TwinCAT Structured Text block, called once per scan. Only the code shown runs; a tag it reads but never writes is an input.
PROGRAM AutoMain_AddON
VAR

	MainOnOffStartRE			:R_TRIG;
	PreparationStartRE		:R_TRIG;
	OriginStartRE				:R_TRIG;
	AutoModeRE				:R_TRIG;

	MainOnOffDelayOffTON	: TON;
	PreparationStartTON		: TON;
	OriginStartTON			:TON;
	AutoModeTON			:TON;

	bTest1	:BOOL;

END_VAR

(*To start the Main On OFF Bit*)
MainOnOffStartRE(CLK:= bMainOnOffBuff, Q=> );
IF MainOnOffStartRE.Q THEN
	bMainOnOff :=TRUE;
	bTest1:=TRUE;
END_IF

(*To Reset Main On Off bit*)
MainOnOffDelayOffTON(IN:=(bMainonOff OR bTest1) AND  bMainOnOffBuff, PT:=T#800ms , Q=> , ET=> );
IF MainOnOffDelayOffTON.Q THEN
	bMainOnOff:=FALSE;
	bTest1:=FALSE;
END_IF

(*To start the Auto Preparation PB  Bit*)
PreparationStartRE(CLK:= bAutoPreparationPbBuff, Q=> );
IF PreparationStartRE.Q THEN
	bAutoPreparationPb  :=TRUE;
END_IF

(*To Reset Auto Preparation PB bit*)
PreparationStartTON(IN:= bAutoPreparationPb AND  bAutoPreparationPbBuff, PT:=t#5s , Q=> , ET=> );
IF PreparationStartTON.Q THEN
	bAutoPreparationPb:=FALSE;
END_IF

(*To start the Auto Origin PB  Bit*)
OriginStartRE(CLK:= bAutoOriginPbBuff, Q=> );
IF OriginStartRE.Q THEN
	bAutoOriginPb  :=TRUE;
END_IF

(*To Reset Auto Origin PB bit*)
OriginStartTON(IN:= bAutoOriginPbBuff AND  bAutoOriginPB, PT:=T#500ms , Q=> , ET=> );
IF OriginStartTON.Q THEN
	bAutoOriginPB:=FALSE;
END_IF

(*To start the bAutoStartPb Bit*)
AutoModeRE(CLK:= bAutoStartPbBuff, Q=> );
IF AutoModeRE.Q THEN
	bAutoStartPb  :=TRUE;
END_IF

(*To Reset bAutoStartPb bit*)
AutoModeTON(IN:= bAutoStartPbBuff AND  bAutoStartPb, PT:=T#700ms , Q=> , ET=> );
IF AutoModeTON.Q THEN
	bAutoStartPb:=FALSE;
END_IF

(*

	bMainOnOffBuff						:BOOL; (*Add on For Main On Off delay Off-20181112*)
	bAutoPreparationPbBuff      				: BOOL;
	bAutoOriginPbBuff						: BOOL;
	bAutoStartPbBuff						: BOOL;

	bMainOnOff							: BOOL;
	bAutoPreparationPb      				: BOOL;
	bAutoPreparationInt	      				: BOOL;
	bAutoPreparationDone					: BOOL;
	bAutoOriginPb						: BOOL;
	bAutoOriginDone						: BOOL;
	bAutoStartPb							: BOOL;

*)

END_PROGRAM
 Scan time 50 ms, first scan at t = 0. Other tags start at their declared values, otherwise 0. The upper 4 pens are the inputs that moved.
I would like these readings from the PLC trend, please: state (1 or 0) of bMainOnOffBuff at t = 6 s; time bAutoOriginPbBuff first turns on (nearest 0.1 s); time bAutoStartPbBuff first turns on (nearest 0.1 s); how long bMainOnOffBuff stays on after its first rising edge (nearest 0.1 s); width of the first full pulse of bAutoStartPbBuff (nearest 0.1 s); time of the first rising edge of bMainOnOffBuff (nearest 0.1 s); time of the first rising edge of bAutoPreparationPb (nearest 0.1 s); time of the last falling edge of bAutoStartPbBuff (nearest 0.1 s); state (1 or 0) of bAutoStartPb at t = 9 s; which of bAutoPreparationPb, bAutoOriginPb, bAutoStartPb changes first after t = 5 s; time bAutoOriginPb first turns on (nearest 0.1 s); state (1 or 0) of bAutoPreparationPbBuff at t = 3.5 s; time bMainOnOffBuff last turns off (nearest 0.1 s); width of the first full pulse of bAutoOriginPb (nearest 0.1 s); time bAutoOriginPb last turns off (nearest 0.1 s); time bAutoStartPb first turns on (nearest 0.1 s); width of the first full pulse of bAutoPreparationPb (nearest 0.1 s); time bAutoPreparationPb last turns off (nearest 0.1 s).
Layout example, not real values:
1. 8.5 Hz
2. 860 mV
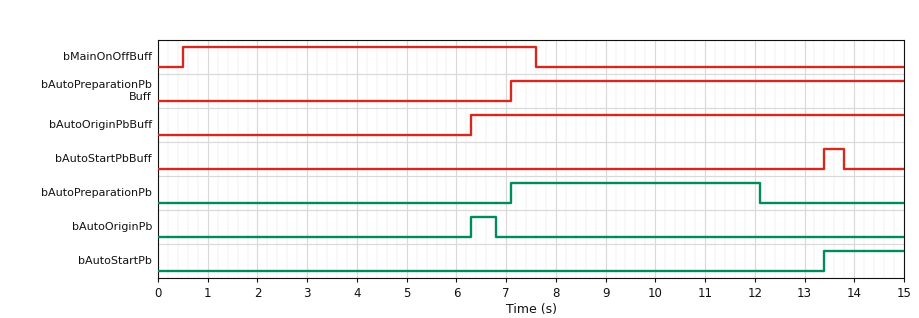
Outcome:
1. 1
2. 6.3 s
3. 13.4 s
4. 7.1 s
5. 0.4 s
6. 0.5 s
7. 7.1 s
8. 13.8 s
9. 0
10. bAutoOriginPb
11. 6.3 s
12. 0
13. 7.6 s
14. 0.5 s
15. 6.8 s
16. 13.4 s
17. 5.0 s
18. 12.1 s
